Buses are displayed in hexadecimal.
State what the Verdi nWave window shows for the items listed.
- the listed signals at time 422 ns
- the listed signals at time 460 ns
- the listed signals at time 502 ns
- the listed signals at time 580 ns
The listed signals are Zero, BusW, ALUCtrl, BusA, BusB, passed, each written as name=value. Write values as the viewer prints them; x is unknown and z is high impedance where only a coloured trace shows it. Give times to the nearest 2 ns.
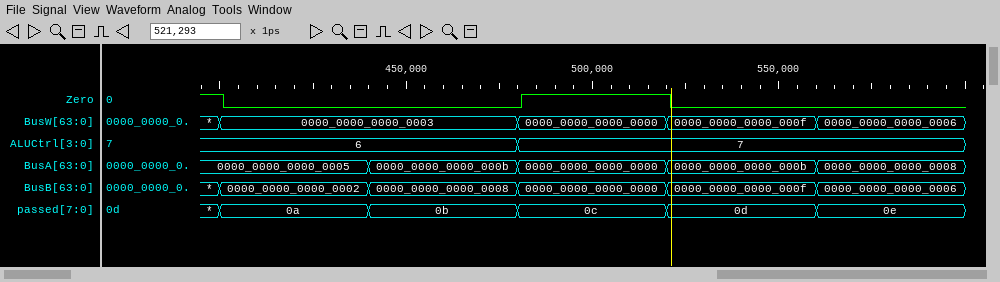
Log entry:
Zero=0, BusW=0000_0000_0000_0003, ALUCtrl=6, BusA=0000_0000_0000_0005, BusB=0000_0000_0000_0002, passed=0a
Zero=0, BusW=0000_0000_0000_0003, ALUCtrl=6, BusA=0000_0000_0000_000b, BusB=0000_0000_0000_0008, passed=0b
Zero=1, BusW=0000_0000_0000_0000, ALUCtrl=7, BusA=0000_0000_0000_0000, BusB=0000_0000_0000_0000, passed=0c
Zero=0, BusW=0000_0000_0000_0006, ALUCtrl=7, BusA=0000_0000_0000_0008, BusB=0000_0000_0000_0006, passed=0e
